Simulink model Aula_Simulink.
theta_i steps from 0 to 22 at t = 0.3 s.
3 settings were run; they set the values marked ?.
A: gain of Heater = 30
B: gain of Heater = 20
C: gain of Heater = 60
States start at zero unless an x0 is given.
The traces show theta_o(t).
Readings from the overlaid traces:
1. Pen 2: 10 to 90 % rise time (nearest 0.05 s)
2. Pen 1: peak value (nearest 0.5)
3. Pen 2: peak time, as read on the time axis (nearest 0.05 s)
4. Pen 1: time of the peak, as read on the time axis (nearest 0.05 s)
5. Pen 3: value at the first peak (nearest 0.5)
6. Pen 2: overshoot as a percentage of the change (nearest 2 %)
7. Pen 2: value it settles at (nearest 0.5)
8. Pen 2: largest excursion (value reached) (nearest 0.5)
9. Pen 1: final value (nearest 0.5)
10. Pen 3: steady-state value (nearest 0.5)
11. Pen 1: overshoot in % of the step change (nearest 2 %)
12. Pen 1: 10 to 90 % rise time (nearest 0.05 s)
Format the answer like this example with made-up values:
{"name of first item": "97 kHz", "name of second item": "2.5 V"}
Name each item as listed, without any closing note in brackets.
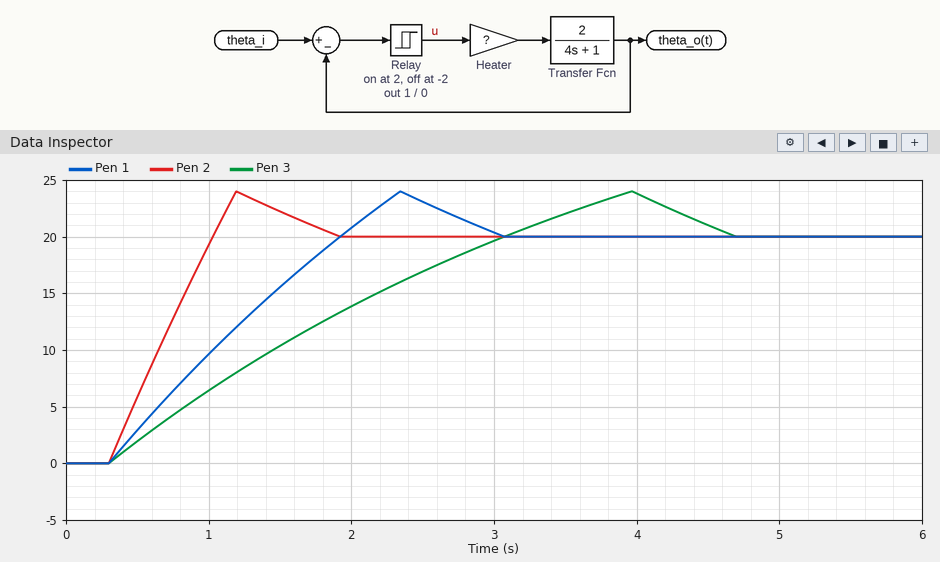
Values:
{"Pen 2: 10 to 90 % rise time": "0.60 s", "Pen 1: peak value": "24.0", "Pen 2: peak time, as read on the time axis": "1.20 s", "Pen 1: time of the peak, as read on the time axis": "2.35 s", "Pen 3: value at the first peak": "24.0", "Pen 2: overshoot as a percentage of the change": "20 %", "Pen 2: value it settles at": "20.0", "Pen 2: largest excursion (value reached)": "24.0", "Pen 1: final value": "20.0", "Pen 3: steady-state value": "20.0", "Pen 1: overshoot in % of the step change": "20 %", "Pen 1: 10 to 90 % rise time": "1.30 s"}
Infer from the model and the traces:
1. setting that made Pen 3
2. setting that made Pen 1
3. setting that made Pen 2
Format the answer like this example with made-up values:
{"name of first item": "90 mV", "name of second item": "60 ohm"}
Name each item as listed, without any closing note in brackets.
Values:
{"setting that made Pen 3": "B", "setting that made Pen 1": "A", "setting that made Pen 2": "C"}
